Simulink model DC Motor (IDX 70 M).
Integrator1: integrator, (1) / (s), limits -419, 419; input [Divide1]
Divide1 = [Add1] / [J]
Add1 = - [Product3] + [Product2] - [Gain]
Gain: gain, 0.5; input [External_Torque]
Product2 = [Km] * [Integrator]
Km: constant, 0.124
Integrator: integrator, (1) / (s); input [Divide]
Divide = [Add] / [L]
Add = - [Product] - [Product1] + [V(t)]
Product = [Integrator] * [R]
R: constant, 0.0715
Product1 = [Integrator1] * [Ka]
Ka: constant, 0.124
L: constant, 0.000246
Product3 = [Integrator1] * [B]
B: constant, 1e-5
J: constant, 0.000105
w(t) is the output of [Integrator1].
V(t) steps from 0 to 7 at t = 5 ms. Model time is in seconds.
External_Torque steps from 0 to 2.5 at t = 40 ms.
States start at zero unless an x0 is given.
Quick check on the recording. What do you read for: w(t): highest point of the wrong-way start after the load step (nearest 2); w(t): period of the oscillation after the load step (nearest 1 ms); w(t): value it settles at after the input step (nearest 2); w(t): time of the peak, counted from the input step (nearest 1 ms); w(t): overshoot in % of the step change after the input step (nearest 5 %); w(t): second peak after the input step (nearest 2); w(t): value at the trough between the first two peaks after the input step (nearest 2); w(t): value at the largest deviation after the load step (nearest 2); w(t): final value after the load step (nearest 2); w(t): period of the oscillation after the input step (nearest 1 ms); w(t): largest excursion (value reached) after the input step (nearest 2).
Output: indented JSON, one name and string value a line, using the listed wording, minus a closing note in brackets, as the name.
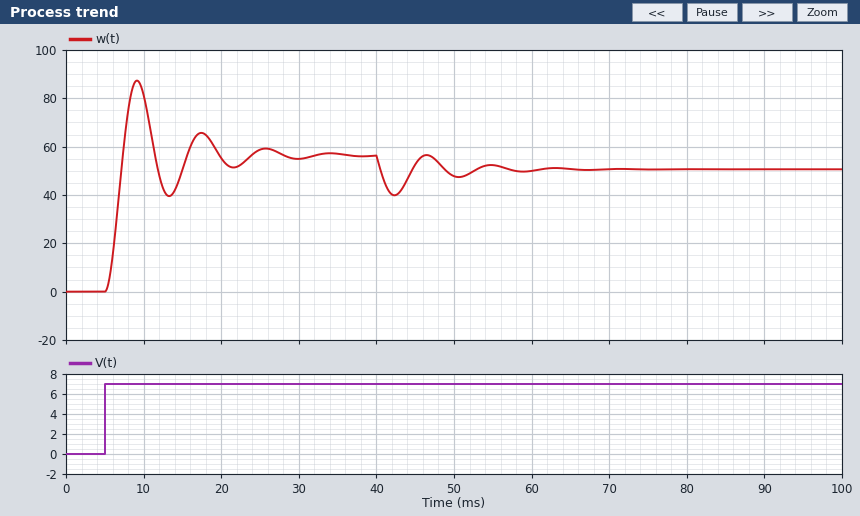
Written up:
{
  "w(t): highest point of the wrong-way start after the load step": "56",
  "w(t): period of the oscillation after the load step": "8 ms",
  "w(t): value it settles at after the input step": "56",
  "w(t): time of the peak, counted from the input step": "4 ms",
  "w(t): overshoot in % of the step change after the input step": "55 %",
  "w(t): second peak after the input step": "66",
  "w(t): value at the trough between the first two peaks after the input step": "40",
  "w(t): value at the largest deviation after the load step": "40",
  "w(t): final value after the load step": "50",
  "w(t): period of the oscillation after the input step": "8 ms",
  "w(t): largest excursion (value reached) after the input step": "88"
}
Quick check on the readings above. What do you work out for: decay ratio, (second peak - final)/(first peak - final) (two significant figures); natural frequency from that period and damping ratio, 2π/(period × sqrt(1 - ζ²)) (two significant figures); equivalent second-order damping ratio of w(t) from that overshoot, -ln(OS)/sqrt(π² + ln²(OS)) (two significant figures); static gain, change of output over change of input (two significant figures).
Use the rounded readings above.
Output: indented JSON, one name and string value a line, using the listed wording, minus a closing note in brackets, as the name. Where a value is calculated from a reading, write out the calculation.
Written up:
{
  "decay ratio, (second peak - final)/(first peak - final)": "(66 - 56) / (88 - 56) = 0.31",
  "natural frequency from that period and damping ratio, 2π/(period × sqrt(1 - ζ²))": "2π / (8 × sqrt(1 - 0.19²)) = 0.80 rad/ms",
  "equivalent second-order damping ratio of w(t) from that overshoot, -ln(OS)/sqrt(π² + ln²(OS))": "ln(0.55) = -0.598; 0.598 / sqrt(9.870 + 0.357) = 0.19",
  "static gain, change of output over change of input": "(56 - 0) / (7 - 0) = 8.0"
}
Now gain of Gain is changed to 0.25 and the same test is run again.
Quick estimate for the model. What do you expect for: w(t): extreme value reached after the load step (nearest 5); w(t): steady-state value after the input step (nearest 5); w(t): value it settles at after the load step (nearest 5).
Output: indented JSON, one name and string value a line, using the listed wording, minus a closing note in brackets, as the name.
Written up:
{
  "w(t): extreme value reached after the load step": "50",
  "w(t): steady-state value after the input step": "55",
  "w(t): value it settles at after the load step": "55"
}
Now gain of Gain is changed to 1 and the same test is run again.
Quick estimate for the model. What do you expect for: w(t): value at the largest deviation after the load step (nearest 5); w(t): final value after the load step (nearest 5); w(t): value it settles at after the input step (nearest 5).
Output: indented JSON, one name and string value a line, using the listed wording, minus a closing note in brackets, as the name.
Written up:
{
  "w(t): value at the largest deviation after the load step": "25",
  "w(t): final value after the load step": "45",
  "w(t): value it settles at after the input step": "55"
}
